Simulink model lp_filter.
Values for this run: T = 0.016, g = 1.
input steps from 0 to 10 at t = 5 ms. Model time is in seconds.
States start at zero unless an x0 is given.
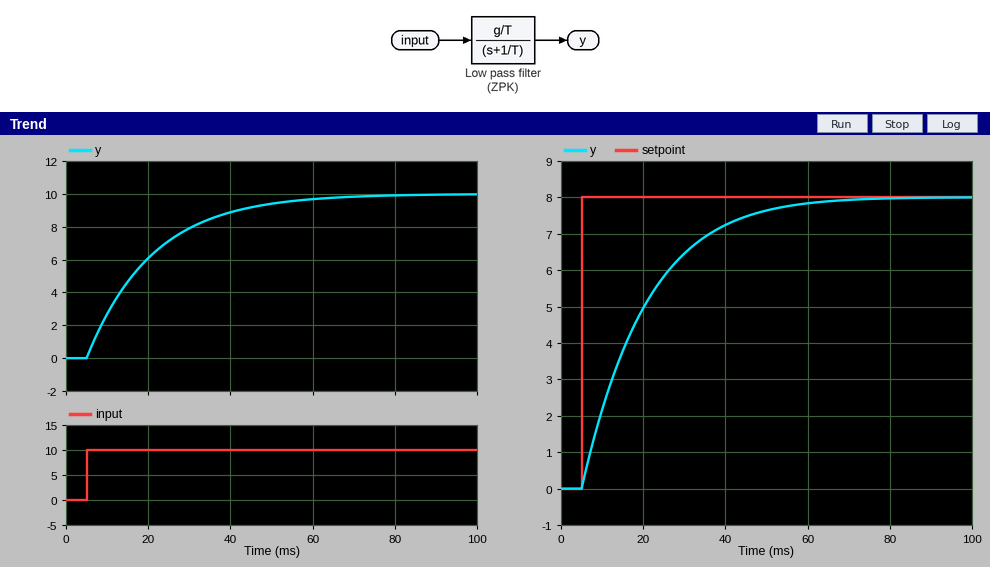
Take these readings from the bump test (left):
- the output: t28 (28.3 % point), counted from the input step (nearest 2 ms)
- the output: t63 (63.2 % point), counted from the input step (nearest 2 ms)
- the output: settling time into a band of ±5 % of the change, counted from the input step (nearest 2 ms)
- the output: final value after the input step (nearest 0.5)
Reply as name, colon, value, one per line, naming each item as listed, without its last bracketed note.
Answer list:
the output: t28 (28.3 % point), counted from the input step: 6 ms
the output: t63 (63.2 % point), counted from the input step: 16 ms
the output: settling time into a band of ±5 % of the change, counted from the input step: 48 ms
the output: final value after the input step: 10.0
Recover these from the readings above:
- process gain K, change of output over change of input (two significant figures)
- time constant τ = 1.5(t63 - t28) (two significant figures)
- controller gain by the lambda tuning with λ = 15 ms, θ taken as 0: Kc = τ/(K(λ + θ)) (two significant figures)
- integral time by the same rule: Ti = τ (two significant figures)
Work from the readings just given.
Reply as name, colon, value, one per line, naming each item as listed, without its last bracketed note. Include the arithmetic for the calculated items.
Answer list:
process gain K, change of output over change of input: (10 - 0) / 10 = 1.0
time constant τ = 1.5(t63 - t28): 1.5 × (16 - 6) = 15 ms
controller gain by the lambda tuning with λ = 15 ms, θ taken as 0: Kc = τ/(K(λ + θ)): 15 / (1 × (15 + 0)) = 1.0
integral time by the same rule: Ti = τ: 15 ms
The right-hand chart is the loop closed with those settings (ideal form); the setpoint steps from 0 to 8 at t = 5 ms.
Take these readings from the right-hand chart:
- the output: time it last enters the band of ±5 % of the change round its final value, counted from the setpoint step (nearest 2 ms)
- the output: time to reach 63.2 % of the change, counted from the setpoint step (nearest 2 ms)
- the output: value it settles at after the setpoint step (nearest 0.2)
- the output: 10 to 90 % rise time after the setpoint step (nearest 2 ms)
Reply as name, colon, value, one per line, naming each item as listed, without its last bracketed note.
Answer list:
the output: time it last enters the band of ±5 % of the change round its final value, counted from the setpoint step: 44 ms
the output: time to reach 63.2 % of the change, counted from the setpoint step: 16 ms
the output: value it settles at after the setpoint step: 8.0
the output: 10 to 90 % rise time after the setpoint step: 32 ms
